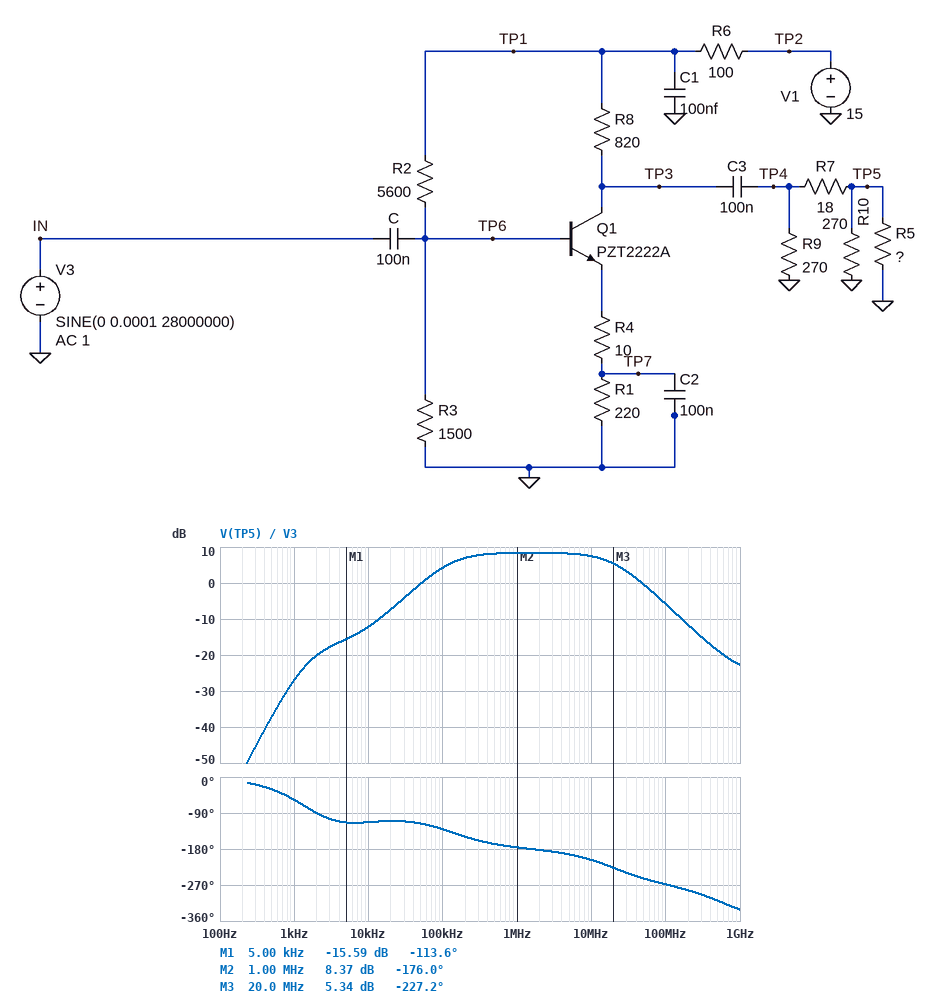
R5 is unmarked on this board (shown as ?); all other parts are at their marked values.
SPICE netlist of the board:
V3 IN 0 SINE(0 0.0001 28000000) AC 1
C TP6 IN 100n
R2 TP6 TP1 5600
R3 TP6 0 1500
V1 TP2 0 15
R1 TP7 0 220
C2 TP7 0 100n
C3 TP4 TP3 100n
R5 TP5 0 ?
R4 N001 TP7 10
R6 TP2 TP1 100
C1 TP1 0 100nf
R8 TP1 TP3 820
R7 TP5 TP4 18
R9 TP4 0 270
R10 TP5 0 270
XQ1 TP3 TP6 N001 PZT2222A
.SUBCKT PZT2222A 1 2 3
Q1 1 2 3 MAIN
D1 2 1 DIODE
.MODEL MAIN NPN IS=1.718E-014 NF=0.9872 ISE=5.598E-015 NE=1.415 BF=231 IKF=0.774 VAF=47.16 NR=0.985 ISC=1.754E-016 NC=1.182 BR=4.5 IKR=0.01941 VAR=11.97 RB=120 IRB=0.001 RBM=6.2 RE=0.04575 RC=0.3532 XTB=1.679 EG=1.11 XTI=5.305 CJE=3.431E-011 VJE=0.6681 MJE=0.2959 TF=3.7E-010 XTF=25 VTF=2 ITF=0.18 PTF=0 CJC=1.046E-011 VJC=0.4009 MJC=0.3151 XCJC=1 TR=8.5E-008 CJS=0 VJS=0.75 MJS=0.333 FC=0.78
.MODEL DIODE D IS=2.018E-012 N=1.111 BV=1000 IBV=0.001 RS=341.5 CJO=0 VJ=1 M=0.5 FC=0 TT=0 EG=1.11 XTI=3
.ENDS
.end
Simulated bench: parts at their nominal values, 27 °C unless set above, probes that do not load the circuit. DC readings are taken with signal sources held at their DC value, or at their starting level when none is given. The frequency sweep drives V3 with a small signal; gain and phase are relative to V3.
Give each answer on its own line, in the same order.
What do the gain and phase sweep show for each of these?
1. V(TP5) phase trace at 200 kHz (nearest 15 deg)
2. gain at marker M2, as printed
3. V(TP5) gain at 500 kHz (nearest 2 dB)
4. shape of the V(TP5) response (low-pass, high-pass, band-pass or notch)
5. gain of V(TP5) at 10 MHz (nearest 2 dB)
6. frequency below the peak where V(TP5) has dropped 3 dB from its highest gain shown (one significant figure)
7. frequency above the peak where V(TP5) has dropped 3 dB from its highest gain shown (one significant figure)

-150 deg
8.37 dB
8 dB
band-pass
8 dB
100 kHz
20 MHz
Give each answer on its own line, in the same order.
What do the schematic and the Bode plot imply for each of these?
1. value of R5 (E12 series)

56 Ω
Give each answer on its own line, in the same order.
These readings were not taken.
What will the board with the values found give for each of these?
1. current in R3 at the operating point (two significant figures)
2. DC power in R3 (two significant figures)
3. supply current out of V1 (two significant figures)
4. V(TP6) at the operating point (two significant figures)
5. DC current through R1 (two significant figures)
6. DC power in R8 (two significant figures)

1.9 mA
5.5 mW
11 mA
2.9 V
9.5 mA
73 mW
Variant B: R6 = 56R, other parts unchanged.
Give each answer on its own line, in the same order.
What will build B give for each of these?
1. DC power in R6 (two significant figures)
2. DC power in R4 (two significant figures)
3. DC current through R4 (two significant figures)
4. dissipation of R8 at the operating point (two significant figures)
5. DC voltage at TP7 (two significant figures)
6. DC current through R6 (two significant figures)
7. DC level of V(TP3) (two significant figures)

7.9 mW
980 µW
9.9 mA
80 mW
2.2 V
12 mA
6.2 V
